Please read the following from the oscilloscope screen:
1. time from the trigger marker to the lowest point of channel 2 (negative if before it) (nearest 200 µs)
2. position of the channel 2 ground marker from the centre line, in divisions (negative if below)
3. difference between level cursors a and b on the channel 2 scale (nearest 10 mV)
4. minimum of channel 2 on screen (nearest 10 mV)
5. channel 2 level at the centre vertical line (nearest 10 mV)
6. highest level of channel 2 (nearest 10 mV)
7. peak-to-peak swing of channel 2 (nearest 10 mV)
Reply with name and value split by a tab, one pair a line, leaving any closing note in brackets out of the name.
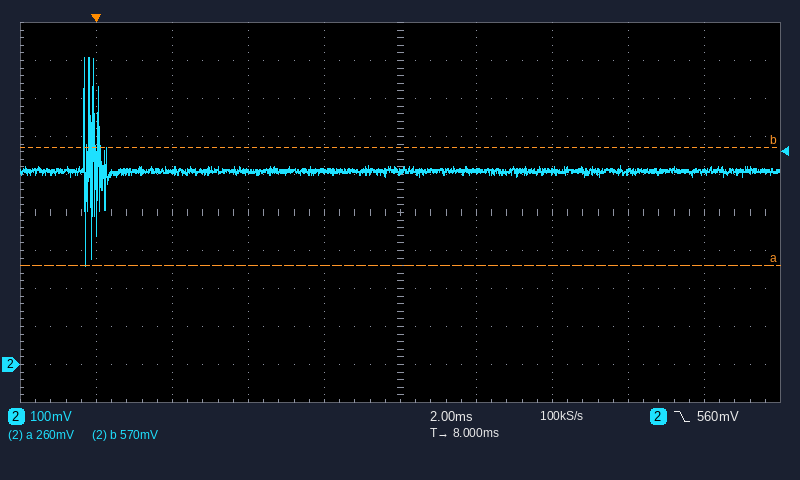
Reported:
time from the trigger marker to the lowest point of channel 2 (negative if before it)	-200 µs
position of the channel 2 ground marker from the centre line, in divisions	-4.0 div
difference between level cursors a and b on the channel 2 scale	310 mV
minimum of channel 2 on screen	260 mV
channel 2 level at the centre vertical line	510 mV
highest level of channel 2	810 mV
peak-to-peak swing of channel 2	550 mV
